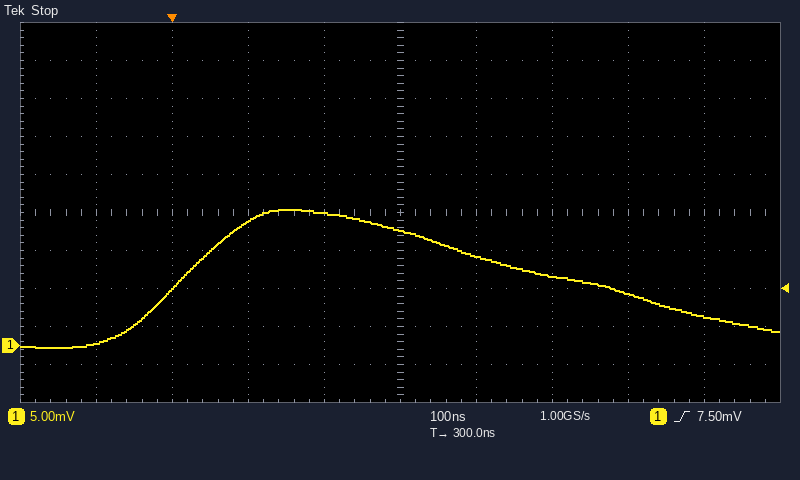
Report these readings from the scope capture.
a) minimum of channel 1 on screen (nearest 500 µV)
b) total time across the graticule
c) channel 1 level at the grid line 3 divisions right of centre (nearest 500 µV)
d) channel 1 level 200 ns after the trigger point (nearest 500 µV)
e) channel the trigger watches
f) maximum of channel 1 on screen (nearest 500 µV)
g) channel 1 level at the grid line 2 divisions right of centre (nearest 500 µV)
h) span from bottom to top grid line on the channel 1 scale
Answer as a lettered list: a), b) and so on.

a) -500 µV
b) 1 µs
c) 7.0 mV
d) 17.5 mV
e) channel 1
f) 18.0 mV
g) 9.0 mV
h) 50 mV
